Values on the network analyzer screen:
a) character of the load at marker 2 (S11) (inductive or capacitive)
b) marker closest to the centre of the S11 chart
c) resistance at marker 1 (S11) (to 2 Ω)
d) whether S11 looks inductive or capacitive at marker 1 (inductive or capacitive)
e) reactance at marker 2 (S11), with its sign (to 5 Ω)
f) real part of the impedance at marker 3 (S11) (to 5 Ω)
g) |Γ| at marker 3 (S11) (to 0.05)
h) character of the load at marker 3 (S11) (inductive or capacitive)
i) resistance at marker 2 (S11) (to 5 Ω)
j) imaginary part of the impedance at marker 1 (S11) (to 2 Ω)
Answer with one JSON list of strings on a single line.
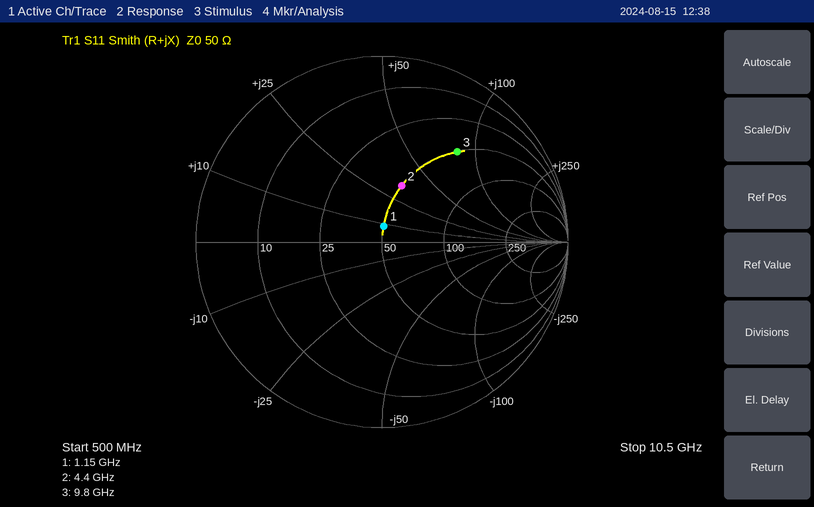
["inductive", "marker 1", "50 Ω", "inductive", "+35 Ω", "50 Ω", "0.65", "inductive", "50 Ω", "+8 Ω"]
